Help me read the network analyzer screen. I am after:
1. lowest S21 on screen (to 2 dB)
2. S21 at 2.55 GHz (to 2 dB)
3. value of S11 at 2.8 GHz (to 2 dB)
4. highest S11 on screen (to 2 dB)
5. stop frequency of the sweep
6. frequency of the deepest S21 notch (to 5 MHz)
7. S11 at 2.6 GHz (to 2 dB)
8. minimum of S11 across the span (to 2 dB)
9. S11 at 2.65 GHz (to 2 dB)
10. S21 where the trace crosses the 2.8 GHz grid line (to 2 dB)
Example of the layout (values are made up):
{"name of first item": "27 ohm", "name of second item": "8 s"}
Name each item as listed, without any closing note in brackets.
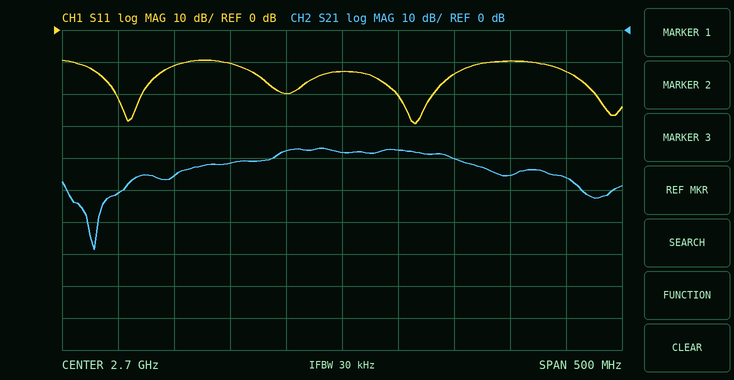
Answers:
{"lowest S21 on screen": "-68 dB", "S21 at 2.55 GHz": "-46 dB", "value of S11 at 2.8 GHz": "-14 dB", "highest S11 on screen": "-10 dB", "stop frequency of the sweep": "2.95 GHz", "frequency of the deepest S21 notch": "2.480 GHz", "S11 at 2.6 GHz": "-10 dB", "minimum of S11 across the span": "-30 dB", "S11 at 2.65 GHz": "-20 dB", "S21 where the trace crosses the 2.8 GHz grid line": "-40 dB"}
